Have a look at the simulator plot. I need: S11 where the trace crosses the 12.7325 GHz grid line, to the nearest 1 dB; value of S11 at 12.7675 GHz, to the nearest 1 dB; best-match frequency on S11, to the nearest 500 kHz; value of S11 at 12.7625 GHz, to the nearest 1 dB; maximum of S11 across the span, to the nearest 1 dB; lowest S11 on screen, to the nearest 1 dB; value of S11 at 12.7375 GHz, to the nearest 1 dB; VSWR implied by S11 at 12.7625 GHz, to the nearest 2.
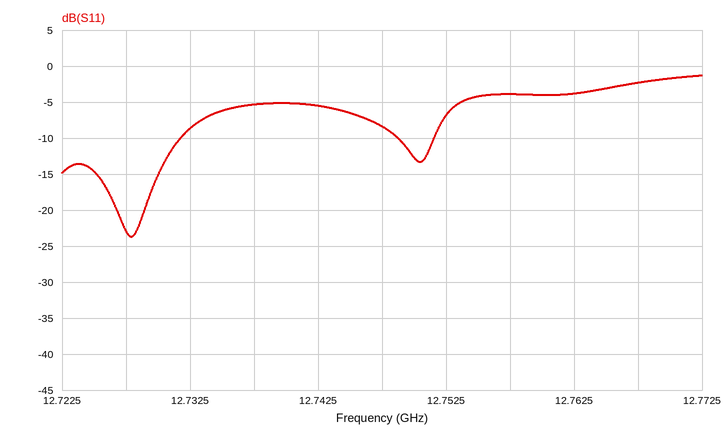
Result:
-9 dB
-2 dB
12.7280 GHz
-4 dB
-1 dB
-24 dB
-5 dB
4
